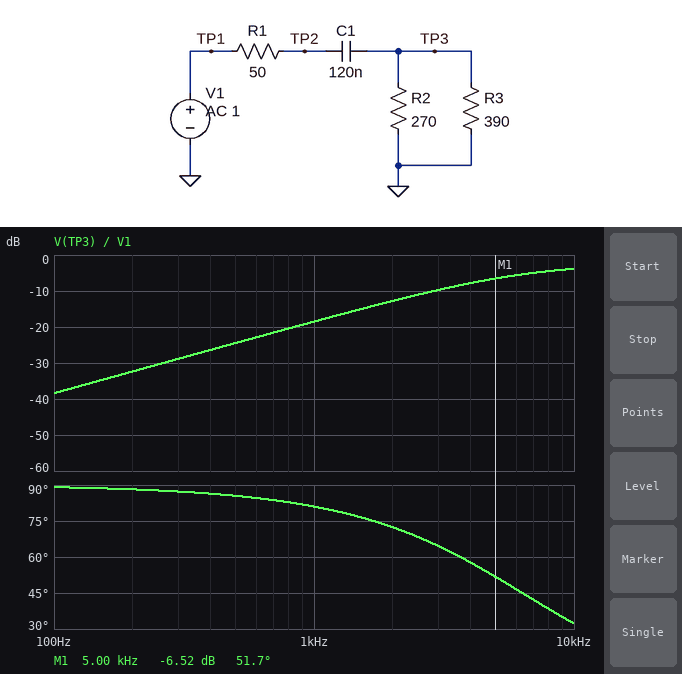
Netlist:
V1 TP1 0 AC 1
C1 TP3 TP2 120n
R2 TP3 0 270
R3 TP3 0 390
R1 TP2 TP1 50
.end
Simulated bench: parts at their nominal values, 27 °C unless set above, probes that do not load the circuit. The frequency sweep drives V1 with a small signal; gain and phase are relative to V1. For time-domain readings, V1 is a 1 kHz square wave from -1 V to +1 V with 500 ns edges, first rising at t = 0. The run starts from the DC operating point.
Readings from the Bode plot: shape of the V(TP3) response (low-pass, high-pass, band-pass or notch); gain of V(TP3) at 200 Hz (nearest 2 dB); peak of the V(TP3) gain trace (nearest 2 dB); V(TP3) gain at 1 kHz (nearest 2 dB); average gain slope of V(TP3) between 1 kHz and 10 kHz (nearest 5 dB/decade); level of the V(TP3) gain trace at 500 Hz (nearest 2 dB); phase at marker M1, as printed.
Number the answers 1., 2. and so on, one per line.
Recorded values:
1. high-pass
2. -32 dB
3. -4 dB
4. -18 dB
5. 15 dB/decade
6. -24 dB
7. 51.7 deg
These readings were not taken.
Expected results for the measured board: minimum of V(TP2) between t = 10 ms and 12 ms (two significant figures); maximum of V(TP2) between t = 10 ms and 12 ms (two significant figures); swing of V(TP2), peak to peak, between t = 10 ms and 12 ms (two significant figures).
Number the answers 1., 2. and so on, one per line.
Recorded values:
1. -1.0 V
2. 1.0 V
3. 2.0 V
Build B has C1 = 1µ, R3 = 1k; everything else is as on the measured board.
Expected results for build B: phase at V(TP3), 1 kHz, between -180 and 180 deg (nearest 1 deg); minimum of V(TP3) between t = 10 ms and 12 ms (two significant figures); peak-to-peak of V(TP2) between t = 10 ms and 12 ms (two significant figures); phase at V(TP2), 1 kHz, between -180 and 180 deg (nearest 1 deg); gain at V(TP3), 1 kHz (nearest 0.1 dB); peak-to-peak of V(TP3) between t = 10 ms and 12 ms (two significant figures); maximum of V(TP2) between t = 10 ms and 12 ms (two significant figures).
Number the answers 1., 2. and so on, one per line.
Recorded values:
1. 31 deg
2. -1.4 V
3. 1.9 V
4. -6 deg
5. -3.2 dB
6. 2.8 V
7. 950 mV
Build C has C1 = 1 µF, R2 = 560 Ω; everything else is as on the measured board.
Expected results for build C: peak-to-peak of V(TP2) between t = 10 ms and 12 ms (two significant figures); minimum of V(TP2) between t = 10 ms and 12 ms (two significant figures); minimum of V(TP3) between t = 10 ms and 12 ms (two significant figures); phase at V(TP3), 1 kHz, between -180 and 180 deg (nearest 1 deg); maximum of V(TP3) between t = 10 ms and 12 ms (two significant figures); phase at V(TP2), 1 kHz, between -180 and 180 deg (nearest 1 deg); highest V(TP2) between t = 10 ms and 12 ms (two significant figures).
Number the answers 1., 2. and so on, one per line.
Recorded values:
1. 1.9 V
2. -950 mV
3. -1.4 V
4. 30 deg
5. 1.4 V
6. -5 deg
7. 950 mV
